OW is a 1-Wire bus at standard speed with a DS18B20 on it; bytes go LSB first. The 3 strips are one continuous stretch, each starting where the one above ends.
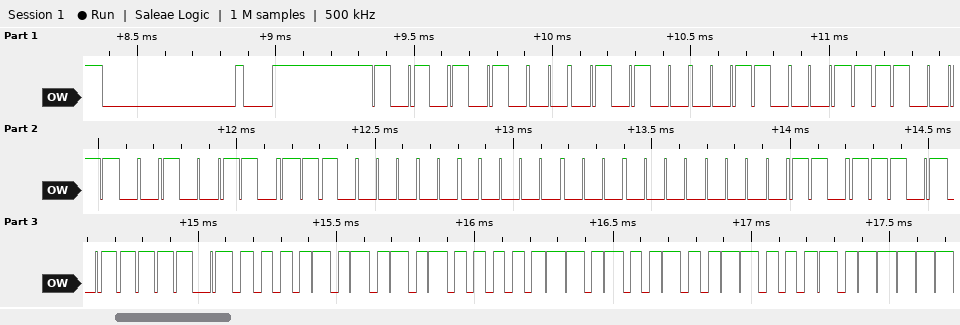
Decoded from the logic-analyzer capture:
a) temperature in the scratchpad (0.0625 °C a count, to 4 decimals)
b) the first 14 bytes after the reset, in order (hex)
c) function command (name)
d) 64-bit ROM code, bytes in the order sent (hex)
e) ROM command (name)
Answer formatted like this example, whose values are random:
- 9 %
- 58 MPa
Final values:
- 85.0000 °C
- 55 28 8C 67 B2 03 00 00 BB BE 50 05 4B 46
- Read Scratchpad
- 28 8C 67 B2 03 00 00 BB
- Match ROM
